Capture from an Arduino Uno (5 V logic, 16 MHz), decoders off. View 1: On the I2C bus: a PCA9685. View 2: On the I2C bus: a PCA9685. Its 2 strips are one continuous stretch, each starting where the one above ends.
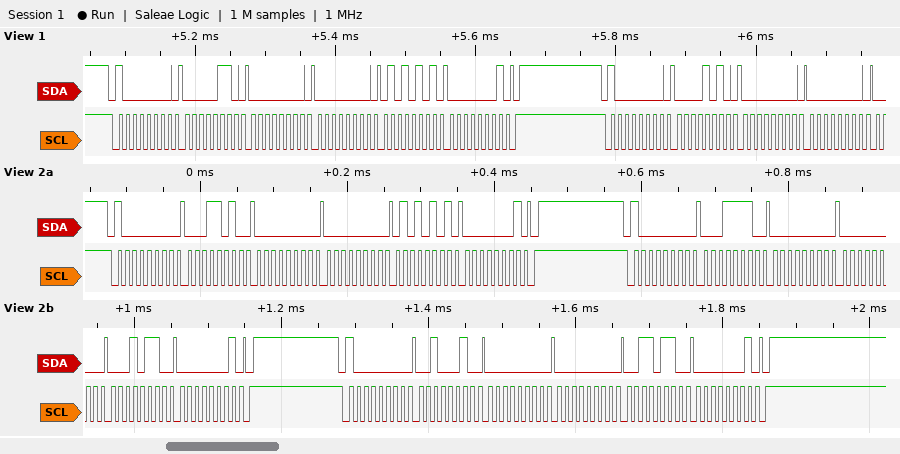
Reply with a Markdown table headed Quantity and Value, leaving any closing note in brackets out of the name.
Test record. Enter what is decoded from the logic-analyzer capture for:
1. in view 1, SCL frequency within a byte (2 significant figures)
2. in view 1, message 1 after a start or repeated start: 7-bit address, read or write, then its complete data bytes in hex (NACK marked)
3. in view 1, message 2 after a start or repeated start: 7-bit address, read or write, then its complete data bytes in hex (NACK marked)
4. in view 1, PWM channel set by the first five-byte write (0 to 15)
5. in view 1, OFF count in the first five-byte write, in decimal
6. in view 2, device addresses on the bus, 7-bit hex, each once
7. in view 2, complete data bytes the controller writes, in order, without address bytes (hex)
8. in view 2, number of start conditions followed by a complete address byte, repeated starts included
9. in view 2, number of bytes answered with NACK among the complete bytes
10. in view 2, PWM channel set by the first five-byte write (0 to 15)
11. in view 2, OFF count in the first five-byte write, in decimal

| Quantity | Value |
|---|---|
| in view 1, SCL frequency within a byte | 100 kHz |
| in view 1, message 1 after a start or repeated start: 7-bit address, read or write, then its complete data bytes in hex | 0x40 write: 06 00 00 55 01 |
| in view 1, message 2 after a start or repeated start: 7-bit address, read or write, then its complete data bytes in hex | 0x40 write: 0A 00 00 |
| in view 1, PWM channel set by the first five-byte write | 0 |
| in view 1, OFF count in the first five-byte write, in decimal | 341 |
| in view 2, device addresses on the bus, 7-bit hex, each once | 0x40 |
| in view 2, complete data bytes the controller writes, in order, without address bytes | 1A 00 00 55 01 1E 00 00 16 01 22 00 00 36 01 |
| in view 2, number of start conditions followed by a complete address byte, repeated starts included | 3 |
| in view 2, number of bytes answered with NACK among the complete bytes | 0 |
| in view 2, PWM channel set by the first five-byte write | 5 |
| in view 2, OFF count in the first five-byte write, in decimal | 341 |
